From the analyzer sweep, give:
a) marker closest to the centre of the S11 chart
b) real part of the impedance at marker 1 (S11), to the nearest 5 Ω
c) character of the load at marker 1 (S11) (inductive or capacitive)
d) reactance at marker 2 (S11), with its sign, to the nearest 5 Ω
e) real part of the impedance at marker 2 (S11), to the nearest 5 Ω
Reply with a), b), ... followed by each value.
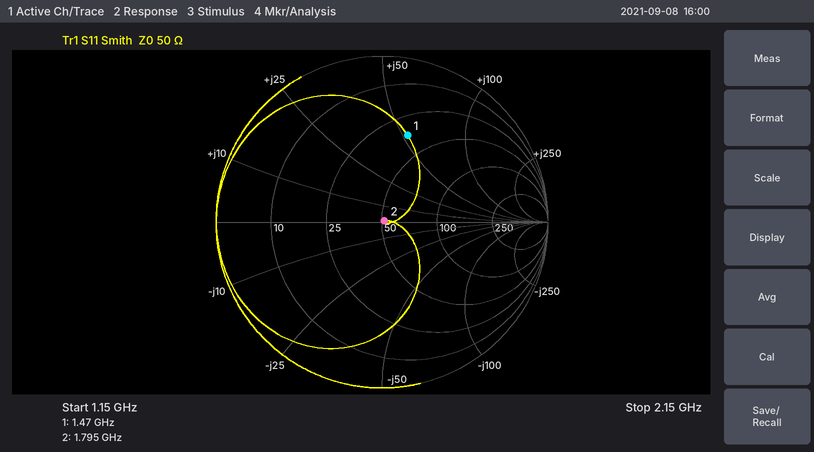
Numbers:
a) marker 2
b) 35 Ω
c) inductive
d) 0 Ω
e) 50 Ω
